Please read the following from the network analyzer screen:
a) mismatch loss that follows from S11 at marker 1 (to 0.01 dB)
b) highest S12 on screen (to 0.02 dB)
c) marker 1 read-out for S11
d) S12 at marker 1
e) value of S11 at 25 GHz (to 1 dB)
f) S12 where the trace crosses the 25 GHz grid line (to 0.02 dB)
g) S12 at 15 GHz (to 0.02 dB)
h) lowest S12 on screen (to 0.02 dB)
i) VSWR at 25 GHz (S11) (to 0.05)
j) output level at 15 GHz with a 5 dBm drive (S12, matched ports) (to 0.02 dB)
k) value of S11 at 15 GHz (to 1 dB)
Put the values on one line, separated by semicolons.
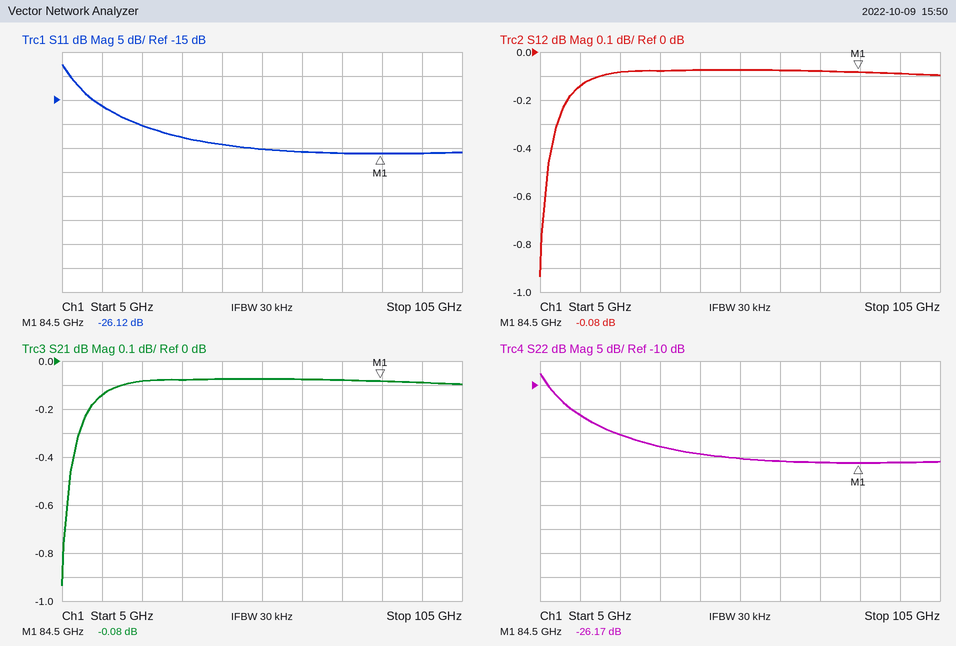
0.01 dB; -0.08 dB; -26.12 dB; -0.08 dB; -20 dB; -0.08 dB; -0.14 dB; -0.94 dB; 1.20; 4.86 dBm; -16 dB
